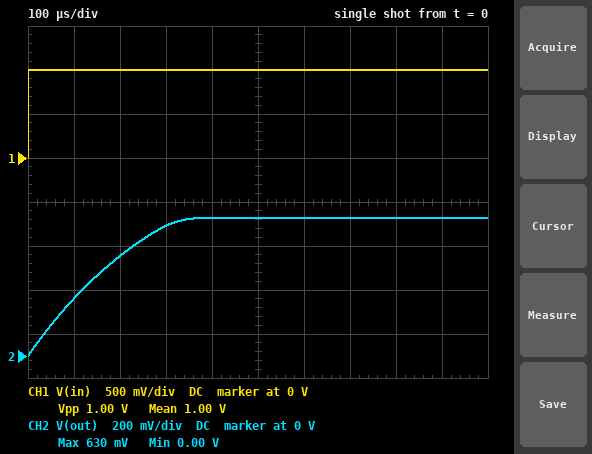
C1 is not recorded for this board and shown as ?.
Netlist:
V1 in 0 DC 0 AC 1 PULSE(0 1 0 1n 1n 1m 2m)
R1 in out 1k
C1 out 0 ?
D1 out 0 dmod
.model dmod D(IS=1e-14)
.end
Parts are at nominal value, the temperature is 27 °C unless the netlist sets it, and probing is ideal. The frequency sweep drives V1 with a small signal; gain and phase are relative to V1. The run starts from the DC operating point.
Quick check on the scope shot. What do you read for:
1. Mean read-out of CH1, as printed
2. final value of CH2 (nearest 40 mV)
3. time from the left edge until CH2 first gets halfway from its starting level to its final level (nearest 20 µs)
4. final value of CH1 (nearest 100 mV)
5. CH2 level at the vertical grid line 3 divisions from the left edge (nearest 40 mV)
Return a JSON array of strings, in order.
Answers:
["1.00 V", "640 mV", "120 µs", "1.0 V", "600 mV"]
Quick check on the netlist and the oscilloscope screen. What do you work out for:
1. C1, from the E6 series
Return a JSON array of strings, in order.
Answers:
["330 nF"]
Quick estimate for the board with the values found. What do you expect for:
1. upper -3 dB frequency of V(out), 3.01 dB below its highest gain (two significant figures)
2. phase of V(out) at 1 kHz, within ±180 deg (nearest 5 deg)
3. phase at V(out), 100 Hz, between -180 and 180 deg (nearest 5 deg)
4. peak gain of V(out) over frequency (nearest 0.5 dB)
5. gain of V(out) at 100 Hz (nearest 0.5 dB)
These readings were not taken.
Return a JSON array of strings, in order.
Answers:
["480 Hz", "-65 deg", "-10 deg", "0 dB", "0 dB"]
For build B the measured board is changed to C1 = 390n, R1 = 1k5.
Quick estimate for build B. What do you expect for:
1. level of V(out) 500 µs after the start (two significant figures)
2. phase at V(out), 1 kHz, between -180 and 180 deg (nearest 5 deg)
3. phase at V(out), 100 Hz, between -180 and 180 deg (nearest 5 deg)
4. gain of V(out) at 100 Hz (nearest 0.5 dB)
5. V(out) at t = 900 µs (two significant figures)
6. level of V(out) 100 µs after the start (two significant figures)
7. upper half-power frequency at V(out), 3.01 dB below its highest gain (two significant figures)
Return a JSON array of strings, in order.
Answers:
["570 mV", "-75 deg", "-20 deg", "-0.5 dB", "620 mV", "160 mV", "270 Hz"]
